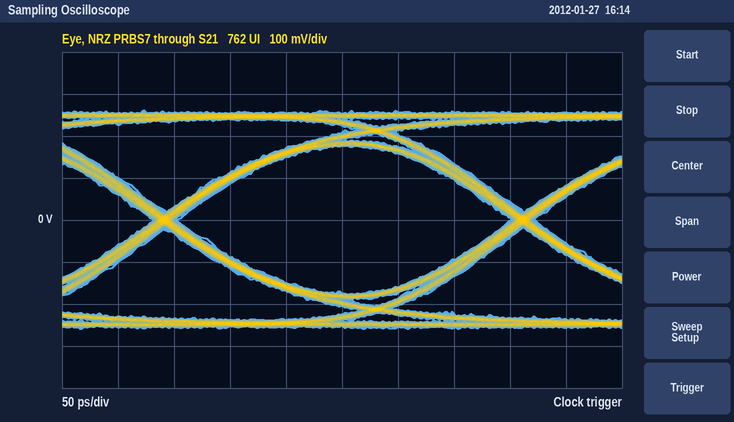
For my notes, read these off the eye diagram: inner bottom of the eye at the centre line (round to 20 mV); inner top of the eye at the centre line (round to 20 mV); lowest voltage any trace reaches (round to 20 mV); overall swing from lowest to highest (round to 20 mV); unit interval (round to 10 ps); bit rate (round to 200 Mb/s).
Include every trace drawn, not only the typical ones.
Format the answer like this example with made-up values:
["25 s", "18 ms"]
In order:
["-180 mV", "180 mV", "-260 mV", "520 mV", "320 ps", "3.2 Gb/s"]
